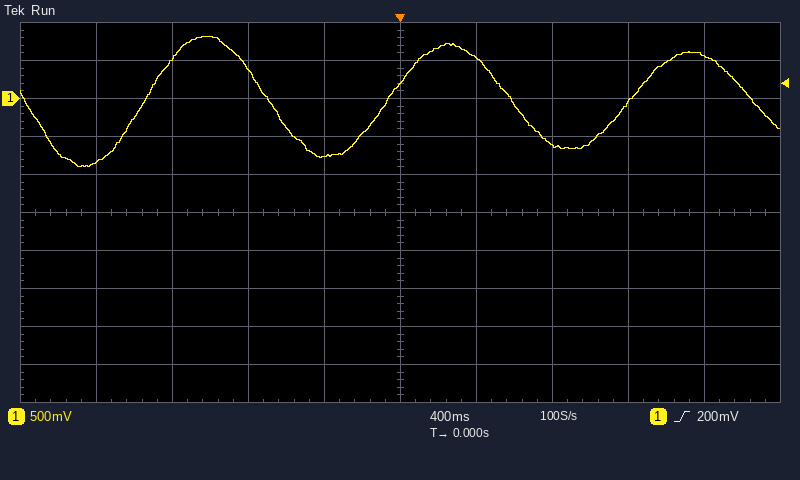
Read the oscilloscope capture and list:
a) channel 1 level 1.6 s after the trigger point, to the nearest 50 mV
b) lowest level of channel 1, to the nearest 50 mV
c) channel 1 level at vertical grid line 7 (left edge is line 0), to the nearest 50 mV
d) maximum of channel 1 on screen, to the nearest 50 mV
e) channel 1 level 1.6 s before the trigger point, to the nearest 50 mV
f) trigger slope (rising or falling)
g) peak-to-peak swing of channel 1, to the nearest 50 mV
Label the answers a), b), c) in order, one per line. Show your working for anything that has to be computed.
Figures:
a) 550 mV
b) -900 mV
c) -600 mV
d) 800 mV
e) -850 mV
f) rising
g) 800 mV − (-900 mV) = 1.70 V
